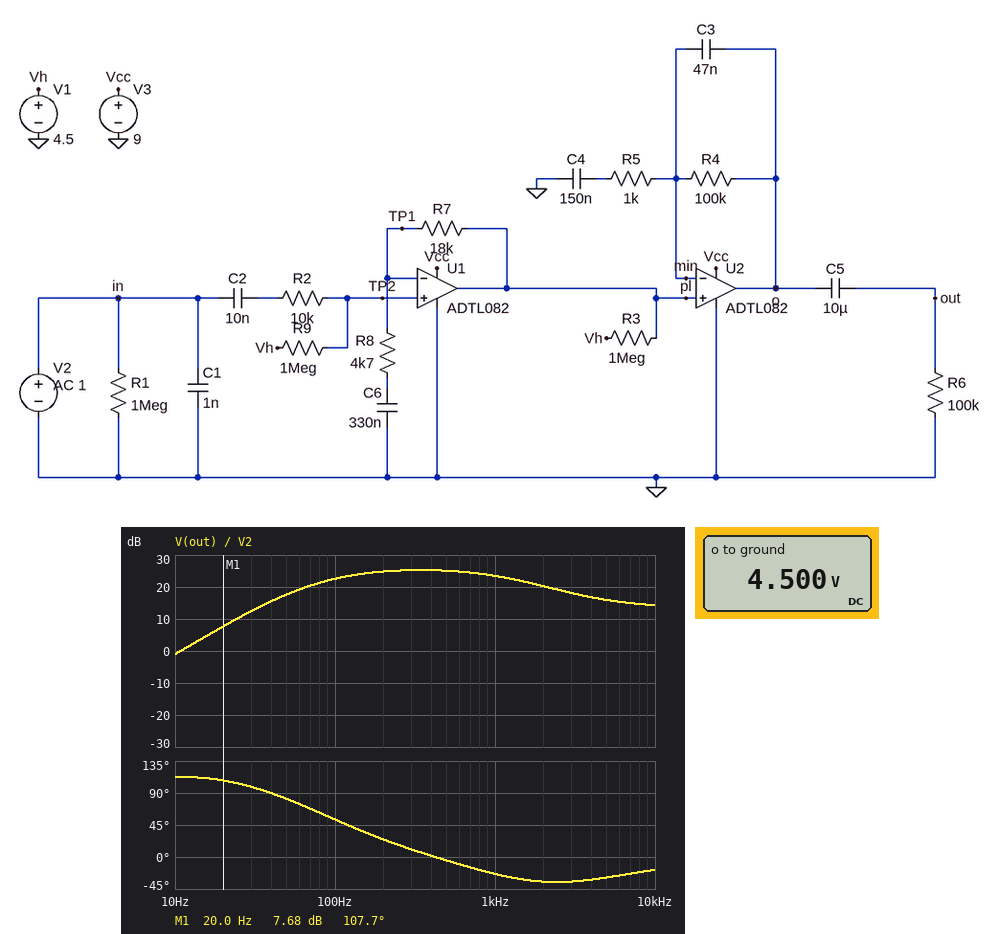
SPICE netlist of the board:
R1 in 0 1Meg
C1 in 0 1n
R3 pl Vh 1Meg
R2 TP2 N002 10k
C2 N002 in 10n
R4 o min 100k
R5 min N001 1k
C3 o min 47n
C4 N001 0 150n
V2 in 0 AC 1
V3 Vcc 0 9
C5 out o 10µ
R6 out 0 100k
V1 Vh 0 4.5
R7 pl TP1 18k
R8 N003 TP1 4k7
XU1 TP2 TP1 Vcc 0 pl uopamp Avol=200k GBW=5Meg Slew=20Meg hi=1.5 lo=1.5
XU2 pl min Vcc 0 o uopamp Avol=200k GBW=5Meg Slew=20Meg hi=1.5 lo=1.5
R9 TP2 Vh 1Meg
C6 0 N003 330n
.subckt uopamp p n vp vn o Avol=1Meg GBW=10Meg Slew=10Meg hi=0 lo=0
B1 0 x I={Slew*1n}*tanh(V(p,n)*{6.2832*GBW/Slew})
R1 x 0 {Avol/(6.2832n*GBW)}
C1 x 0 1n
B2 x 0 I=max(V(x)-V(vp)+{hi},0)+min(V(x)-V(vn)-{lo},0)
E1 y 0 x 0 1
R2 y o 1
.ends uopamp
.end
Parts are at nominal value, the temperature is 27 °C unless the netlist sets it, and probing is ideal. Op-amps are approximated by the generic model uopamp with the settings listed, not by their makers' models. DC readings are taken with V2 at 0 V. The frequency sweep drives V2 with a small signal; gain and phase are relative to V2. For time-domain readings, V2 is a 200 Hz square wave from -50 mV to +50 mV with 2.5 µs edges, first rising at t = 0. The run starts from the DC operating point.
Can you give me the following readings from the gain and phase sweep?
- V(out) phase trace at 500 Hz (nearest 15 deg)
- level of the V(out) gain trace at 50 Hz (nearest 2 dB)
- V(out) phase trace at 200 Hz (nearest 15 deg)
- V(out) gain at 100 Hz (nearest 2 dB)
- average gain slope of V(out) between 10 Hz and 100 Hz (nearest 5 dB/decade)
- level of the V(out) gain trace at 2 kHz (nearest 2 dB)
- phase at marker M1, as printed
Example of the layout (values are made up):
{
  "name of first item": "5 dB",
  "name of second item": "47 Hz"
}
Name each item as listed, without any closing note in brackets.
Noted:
{
  "V(out) phase trace at 500 Hz": "0 deg",
  "level of the V(out) gain trace at 50 Hz": "18 dB",
  "V(out) phase trace at 200 Hz": "30 deg",
  "V(out) gain at 100 Hz": "22 dB",
  "average gain slope of V(out) between 10 Hz and 100 Hz": "25 dB/decade",
  "level of the V(out) gain trace at 2 kHz": "20 dB",
  "phase at marker M1, as printed": "107.7 deg"
}
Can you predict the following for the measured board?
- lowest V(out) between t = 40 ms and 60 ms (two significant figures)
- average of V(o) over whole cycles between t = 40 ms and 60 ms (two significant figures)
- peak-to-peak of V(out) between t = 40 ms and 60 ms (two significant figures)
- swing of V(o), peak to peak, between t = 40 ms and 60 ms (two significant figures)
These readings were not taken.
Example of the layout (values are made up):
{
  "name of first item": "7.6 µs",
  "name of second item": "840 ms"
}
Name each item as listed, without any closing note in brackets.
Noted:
{
  "lowest V(out) between t = 40 ms and 60 ms": "-1.4 V",
  "average of V(o) over whole cycles between t = 40 ms and 60 ms": "4.5 V",
  "peak-to-peak of V(out) between t = 40 ms and 60 ms": "2.7 V",
  "swing of V(o), peak to peak, between t = 40 ms and 60 ms": "2.7 V"
}
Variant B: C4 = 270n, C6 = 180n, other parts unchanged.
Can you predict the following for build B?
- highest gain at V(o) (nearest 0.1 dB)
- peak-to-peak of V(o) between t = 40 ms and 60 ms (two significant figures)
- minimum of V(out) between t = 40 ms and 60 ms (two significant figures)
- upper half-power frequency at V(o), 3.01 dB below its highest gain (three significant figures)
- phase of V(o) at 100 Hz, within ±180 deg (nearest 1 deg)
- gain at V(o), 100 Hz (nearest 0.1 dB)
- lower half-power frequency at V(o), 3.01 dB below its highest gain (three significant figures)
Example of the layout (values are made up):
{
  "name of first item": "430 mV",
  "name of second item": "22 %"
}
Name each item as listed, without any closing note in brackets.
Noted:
{
  "highest gain at V(o)": "27.9 dB",
  "peak-to-peak of V(o) between t = 40 ms and 60 ms": "3.6 V",
  "minimum of V(out) between t = 40 ms and 60 ms": "-1.8 V",
  "upper half-power frequency at V(o), 3.01 dB below its highest gain": "931 Hz",
  "phase of V(o) at 100 Hz, within ±180 deg": "57 deg",
  "gain at V(o), 100 Hz": "23.6 dB",
  "lower half-power frequency at V(o), 3.01 dB below its highest gain": "123 Hz"
}
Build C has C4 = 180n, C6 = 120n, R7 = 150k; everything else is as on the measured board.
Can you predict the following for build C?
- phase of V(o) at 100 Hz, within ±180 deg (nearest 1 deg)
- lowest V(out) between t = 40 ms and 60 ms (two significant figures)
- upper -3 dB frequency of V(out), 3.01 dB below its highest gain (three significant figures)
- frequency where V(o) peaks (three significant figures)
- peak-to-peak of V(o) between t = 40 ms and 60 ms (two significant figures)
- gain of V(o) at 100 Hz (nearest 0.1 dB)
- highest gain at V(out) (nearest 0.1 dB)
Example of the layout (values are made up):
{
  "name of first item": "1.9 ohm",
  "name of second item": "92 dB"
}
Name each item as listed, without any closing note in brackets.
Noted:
{
  "phase of V(o) at 100 Hz, within ±180 deg": "84 deg",
  "lowest V(out) between t = 40 ms and 60 ms": "-3.0 V",
  "upper -3 dB frequency of V(out), 3.01 dB below its highest gain": "1.45 kHz",
  "frequency where V(o) peaks": "513 Hz",
  "peak-to-peak of V(o) between t = 40 ms and 60 ms": "6.0 V",
  "gain of V(o) at 100 Hz": "33.9 dB",
  "highest gain at V(out)": "41.6 dB"
}
